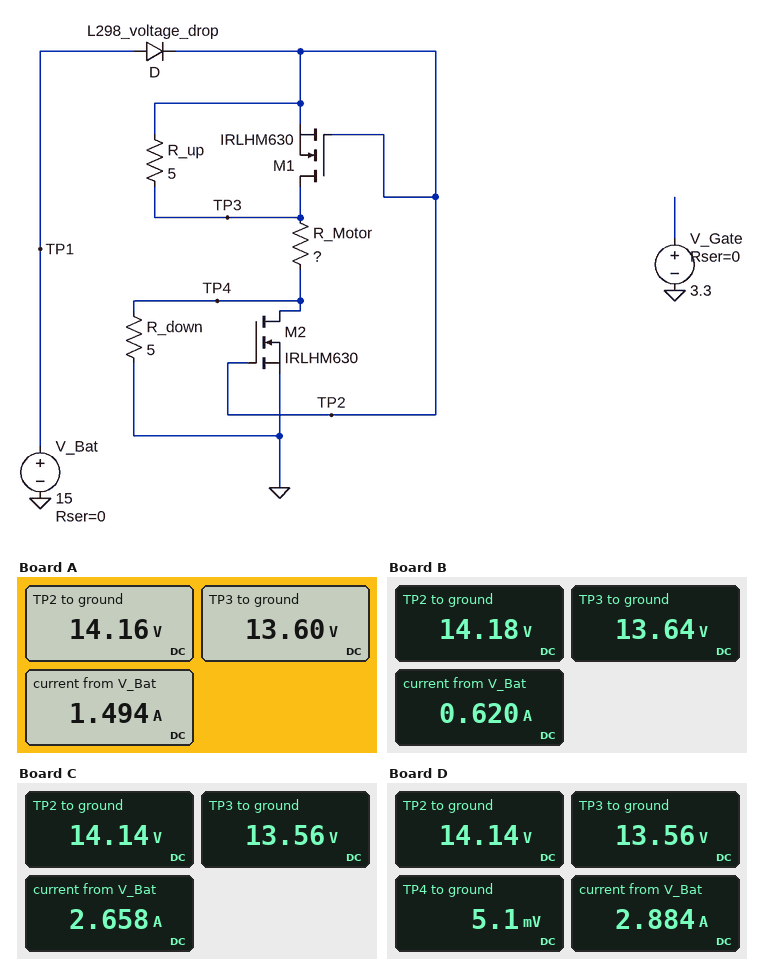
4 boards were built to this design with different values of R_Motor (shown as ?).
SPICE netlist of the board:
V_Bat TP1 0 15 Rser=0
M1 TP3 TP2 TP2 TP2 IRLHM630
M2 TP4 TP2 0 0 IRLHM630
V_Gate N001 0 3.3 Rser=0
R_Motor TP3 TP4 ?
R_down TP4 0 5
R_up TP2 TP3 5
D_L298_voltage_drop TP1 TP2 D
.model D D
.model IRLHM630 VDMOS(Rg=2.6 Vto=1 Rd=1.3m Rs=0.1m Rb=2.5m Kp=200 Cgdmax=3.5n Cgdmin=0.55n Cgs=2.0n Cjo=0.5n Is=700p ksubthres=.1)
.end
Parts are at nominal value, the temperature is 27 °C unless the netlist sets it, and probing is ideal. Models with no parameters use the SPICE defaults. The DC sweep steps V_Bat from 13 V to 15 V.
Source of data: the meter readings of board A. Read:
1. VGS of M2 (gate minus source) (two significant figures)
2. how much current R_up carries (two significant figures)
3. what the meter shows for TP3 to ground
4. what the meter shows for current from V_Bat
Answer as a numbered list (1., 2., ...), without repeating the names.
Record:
1. 14 V
2. 110 mA
3. 13.60 V
4. 1.494 A
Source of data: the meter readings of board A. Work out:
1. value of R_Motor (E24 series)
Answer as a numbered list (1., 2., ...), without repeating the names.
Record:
1. 9.1 Ω
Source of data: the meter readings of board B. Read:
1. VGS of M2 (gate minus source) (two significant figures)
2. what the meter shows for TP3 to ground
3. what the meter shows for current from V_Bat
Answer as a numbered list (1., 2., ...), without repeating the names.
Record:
1. 14 V
2. 13.64 V
3. 0.620 A
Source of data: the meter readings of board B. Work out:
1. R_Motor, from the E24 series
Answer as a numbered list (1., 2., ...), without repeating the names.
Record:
1. 22 Ω
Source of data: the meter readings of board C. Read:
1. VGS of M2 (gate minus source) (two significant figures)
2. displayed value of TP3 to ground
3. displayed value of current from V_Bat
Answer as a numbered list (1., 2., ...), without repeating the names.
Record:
1. 14 V
2. 13.56 V
3. 2.658 A
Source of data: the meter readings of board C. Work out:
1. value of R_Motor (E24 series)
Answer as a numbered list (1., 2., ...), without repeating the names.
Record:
1. 5.1 Ω
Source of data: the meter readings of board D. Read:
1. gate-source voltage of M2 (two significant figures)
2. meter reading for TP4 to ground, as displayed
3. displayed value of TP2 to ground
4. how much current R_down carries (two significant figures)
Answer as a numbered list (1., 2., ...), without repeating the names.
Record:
1. 14 V
2. 5.1 mV
3. 14.14 V
4. 1.0 mA
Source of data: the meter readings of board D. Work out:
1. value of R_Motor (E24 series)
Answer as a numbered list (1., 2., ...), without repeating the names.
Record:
1. 4.7 Ω
